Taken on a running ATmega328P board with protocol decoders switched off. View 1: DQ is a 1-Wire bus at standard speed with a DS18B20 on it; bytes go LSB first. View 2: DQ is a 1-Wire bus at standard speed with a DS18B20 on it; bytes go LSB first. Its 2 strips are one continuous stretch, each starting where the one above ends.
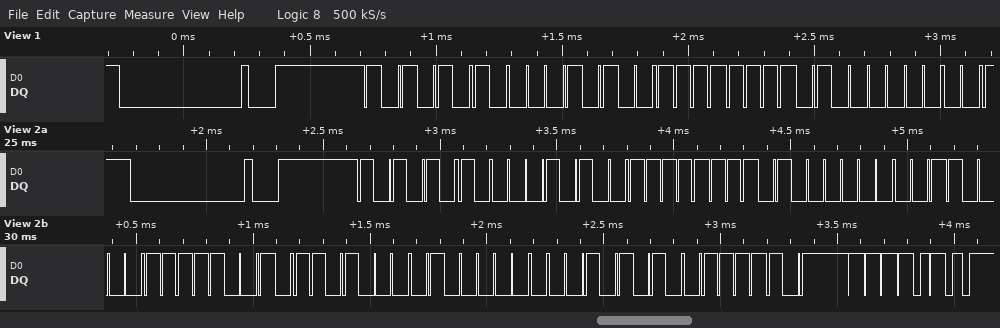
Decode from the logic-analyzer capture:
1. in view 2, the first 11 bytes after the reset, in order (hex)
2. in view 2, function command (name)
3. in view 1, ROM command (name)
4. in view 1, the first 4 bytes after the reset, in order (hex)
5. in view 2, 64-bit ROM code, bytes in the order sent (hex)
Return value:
55 28 FF 02 0C 9F 16 02 54 BE 2F
Read Scratchpad
Match ROM
55 28 FF 02
28 FF 02 0C 9F 16 02 54
